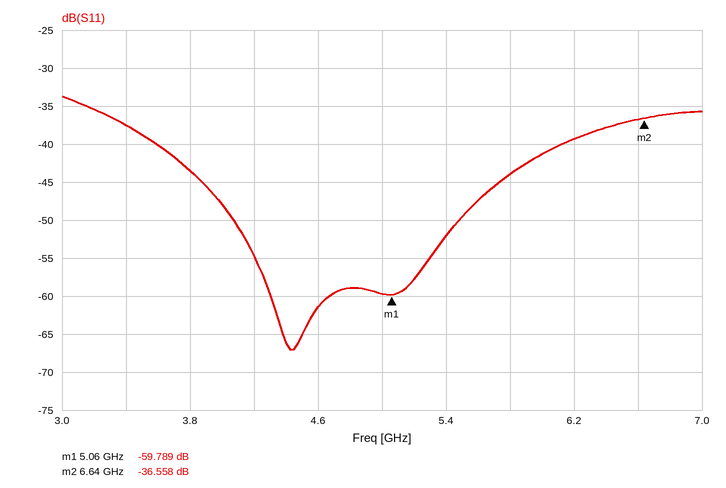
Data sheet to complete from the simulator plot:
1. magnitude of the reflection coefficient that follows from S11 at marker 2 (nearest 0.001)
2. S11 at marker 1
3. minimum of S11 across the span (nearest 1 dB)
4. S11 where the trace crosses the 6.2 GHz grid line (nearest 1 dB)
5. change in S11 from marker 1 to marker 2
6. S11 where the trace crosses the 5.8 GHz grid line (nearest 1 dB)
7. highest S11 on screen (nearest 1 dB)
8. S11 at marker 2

0.015
-59.789 dB
-67 dB
-39 dB
23.231 dB
-44 dB
-34 dB
-36.558 dB
